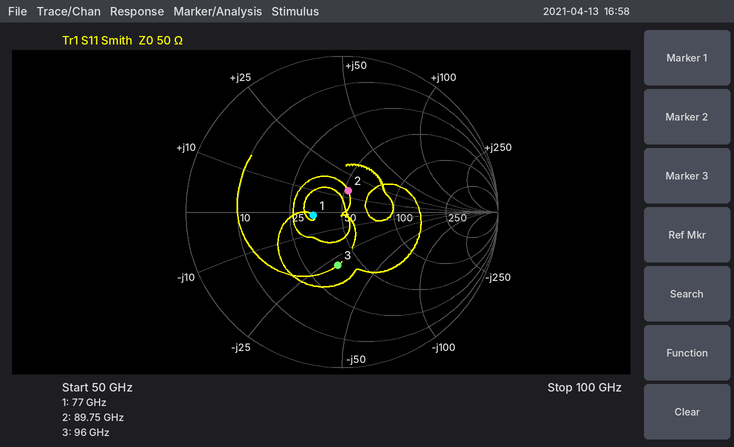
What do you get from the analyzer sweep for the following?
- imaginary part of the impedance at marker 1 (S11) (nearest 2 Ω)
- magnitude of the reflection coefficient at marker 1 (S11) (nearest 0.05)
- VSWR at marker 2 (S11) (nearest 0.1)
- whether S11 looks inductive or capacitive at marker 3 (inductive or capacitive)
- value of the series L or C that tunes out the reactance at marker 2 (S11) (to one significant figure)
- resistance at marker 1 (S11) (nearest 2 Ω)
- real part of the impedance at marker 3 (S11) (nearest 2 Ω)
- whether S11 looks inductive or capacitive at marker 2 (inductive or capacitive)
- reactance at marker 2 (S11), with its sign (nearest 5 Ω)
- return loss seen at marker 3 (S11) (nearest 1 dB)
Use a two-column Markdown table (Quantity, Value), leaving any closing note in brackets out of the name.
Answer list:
| Quantity | Value |
|---|---|
| imaginary part of the impedance at marker 1 (S11) | -2 Ω |
| magnitude of the reflection coefficient at marker 1 (S11) | 0.20 |
| VSWR at marker 2 (S11) | 1.3 |
| whether S11 looks inductive or capacitive at marker 3 | capacitive |
| value of the series L or C that tunes out the reactance at marker 2 (S11) | 100 fF |
| resistance at marker 1 (S11) | 34 Ω |
| real part of the impedance at marker 3 (S11) | 38 Ω |
| whether S11 looks inductive or capacitive at marker 2 | inductive |
| reactance at marker 2 (S11), with its sign | +15 Ω |
| return loss seen at marker 3 (S11) | 9 dB |
